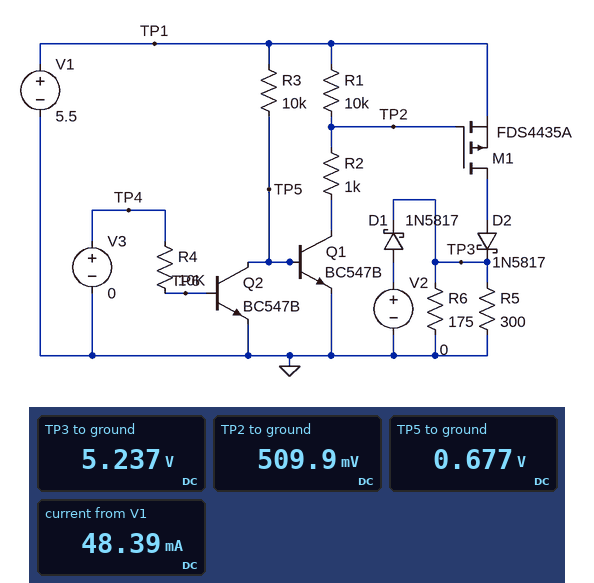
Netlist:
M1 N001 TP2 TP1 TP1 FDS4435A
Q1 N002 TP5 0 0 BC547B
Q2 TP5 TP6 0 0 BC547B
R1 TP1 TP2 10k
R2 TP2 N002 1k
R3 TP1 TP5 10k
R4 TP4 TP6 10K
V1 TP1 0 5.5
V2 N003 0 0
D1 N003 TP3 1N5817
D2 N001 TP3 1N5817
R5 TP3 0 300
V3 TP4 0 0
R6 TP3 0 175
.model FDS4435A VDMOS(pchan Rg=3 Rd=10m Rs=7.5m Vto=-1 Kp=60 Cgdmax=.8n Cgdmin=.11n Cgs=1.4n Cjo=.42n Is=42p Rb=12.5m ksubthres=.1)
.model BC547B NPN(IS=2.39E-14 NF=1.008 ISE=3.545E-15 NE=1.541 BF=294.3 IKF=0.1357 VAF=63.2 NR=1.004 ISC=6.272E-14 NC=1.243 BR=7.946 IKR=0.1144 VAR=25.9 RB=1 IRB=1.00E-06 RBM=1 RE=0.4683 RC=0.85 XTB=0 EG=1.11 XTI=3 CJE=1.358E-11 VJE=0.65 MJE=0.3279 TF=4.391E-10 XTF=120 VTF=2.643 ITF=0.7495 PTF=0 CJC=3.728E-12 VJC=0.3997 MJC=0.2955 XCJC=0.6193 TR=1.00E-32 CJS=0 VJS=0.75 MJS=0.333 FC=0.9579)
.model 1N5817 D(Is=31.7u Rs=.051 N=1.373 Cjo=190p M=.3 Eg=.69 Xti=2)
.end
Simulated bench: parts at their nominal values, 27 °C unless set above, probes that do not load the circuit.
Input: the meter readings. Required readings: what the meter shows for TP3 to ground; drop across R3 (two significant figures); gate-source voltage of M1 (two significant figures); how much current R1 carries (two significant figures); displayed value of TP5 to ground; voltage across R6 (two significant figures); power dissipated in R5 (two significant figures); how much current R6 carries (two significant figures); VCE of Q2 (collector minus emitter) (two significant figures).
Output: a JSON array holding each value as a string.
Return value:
["5.237 V", "4.8 V", "-5.0 V", "500 µA", "0.677 V", "5.2 V", "91 mW", "30 mA", "680 mV"]
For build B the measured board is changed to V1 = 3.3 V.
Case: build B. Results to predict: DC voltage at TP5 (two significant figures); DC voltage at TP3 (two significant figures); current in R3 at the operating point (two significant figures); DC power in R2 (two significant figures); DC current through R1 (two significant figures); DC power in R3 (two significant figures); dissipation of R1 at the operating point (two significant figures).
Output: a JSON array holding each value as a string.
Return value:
["660 mV", "3.1 V", "260 µA", "89 µW", "300 µA", "700 µW", "890 µW"]
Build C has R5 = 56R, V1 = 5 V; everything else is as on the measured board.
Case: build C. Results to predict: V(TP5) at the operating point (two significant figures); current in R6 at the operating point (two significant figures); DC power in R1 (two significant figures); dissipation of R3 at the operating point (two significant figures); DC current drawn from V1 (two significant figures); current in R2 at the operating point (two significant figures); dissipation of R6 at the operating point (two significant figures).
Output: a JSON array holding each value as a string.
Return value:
["670 mV", "27 mA", "2.1 mW", "1.9 mW", "110 mA", "450 µA", "130 mW"]
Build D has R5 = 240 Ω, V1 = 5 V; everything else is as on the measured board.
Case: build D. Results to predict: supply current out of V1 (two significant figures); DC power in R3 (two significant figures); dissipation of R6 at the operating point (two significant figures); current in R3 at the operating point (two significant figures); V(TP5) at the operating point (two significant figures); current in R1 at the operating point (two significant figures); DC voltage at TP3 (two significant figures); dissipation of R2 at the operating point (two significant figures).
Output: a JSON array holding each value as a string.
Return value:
["48 mA", "1.9 mW", "130 mW", "430 µA", "670 mV", "450 µA", "4.7 V", "210 µW"]
